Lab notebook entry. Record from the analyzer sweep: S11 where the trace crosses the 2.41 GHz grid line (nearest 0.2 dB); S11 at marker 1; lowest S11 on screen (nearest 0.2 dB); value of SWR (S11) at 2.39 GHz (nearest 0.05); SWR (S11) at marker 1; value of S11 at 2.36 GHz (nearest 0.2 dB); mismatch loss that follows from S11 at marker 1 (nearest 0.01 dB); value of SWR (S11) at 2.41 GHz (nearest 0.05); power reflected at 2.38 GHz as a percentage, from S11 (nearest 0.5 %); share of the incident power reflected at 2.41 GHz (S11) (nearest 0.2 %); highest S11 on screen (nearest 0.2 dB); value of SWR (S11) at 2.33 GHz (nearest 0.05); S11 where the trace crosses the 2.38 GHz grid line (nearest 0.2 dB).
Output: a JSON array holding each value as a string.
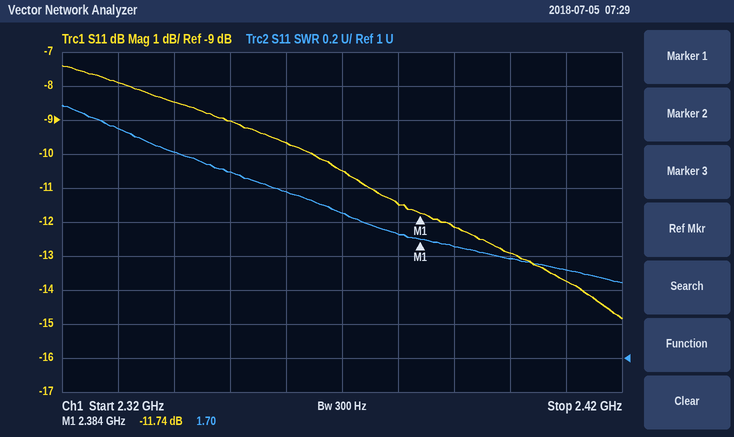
["-13.8 dB", "-11.74 dB", "-14.8 dB", "1.65", "1.70", "-9.6 dB", "0.30 dB", "1.50", "7.0 %", "4.2 %", "-7.4 dB", "2.35", "-11.4 dB"]
